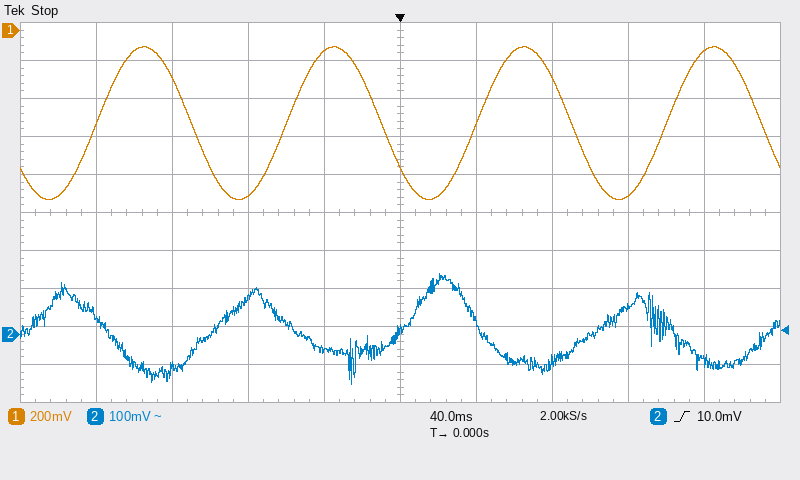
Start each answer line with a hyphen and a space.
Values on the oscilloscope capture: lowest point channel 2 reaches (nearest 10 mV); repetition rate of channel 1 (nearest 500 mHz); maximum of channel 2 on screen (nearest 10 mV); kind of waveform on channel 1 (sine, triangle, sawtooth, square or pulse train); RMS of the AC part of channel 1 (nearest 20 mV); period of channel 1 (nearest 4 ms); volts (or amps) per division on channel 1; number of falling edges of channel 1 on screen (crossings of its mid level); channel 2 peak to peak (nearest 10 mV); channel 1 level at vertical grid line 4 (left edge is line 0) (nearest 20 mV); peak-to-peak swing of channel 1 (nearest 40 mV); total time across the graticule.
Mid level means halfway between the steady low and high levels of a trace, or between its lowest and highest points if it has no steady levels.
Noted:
- -130 mV
- 10.0 Hz
- 160 mV
- sine
- 280 mV
- 100 ms
- 200 mV
- 4
- 290 mV
- -120 mV
- 800 mV
- 400 ms
